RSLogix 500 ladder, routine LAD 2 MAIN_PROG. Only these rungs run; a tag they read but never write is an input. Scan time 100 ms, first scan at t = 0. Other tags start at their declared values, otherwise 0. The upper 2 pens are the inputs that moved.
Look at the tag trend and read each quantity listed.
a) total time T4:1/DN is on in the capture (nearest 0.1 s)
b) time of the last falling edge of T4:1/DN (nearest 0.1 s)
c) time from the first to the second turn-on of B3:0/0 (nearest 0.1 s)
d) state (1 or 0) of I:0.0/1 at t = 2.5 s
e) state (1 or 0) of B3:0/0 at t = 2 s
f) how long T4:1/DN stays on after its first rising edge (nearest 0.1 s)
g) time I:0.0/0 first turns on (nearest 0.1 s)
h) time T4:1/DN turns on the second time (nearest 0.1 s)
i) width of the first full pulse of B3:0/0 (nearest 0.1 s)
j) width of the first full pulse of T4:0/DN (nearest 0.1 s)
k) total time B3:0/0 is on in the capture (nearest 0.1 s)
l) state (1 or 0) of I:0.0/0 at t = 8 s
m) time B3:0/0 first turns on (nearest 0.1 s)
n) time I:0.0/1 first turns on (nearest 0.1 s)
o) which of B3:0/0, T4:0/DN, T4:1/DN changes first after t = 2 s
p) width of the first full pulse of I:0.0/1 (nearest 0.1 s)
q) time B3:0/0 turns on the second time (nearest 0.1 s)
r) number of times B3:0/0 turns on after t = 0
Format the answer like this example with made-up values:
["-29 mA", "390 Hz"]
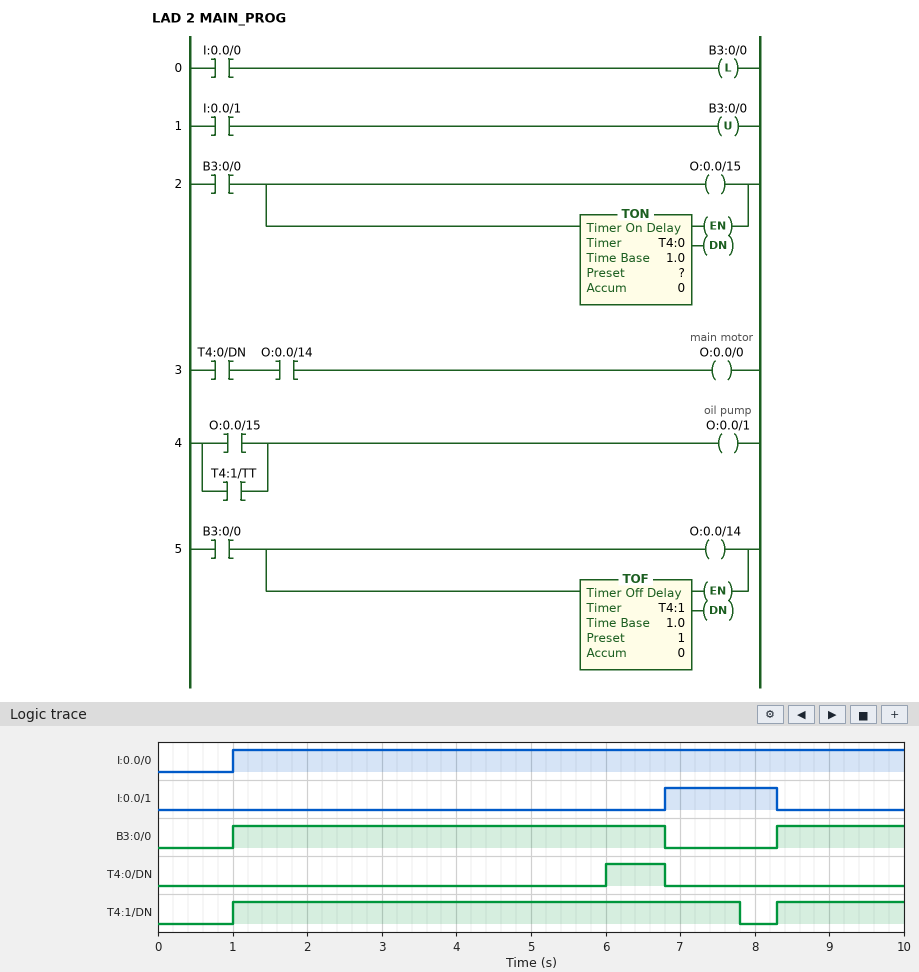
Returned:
["8.5 s", "7.8 s", "7.3 s", "0", "1", "6.8 s", "1.0 s", "8.3 s", "5.8 s", "0.8 s", "7.5 s", "1", "1.0 s", "6.8 s", "T4:0/DN", "1.5 s", "8.3 s", "2"]
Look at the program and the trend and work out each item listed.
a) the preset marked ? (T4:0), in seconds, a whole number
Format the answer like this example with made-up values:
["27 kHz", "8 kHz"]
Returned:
["5 s"]
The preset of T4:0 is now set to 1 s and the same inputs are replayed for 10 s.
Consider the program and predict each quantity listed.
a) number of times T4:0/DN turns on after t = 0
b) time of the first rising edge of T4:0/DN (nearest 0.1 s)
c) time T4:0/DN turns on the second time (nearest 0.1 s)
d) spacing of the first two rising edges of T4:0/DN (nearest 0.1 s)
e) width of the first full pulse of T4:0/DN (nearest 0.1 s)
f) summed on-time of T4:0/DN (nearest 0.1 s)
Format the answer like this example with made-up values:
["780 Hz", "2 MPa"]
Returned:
["2", "2.0 s", "9.3 s", "7.3 s", "4.8 s", "5.5 s"]
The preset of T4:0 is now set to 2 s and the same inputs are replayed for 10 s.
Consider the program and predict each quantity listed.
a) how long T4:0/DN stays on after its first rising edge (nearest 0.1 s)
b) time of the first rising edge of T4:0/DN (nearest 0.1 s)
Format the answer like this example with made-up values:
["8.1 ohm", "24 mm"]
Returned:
["3.8 s", "3.0 s"]
